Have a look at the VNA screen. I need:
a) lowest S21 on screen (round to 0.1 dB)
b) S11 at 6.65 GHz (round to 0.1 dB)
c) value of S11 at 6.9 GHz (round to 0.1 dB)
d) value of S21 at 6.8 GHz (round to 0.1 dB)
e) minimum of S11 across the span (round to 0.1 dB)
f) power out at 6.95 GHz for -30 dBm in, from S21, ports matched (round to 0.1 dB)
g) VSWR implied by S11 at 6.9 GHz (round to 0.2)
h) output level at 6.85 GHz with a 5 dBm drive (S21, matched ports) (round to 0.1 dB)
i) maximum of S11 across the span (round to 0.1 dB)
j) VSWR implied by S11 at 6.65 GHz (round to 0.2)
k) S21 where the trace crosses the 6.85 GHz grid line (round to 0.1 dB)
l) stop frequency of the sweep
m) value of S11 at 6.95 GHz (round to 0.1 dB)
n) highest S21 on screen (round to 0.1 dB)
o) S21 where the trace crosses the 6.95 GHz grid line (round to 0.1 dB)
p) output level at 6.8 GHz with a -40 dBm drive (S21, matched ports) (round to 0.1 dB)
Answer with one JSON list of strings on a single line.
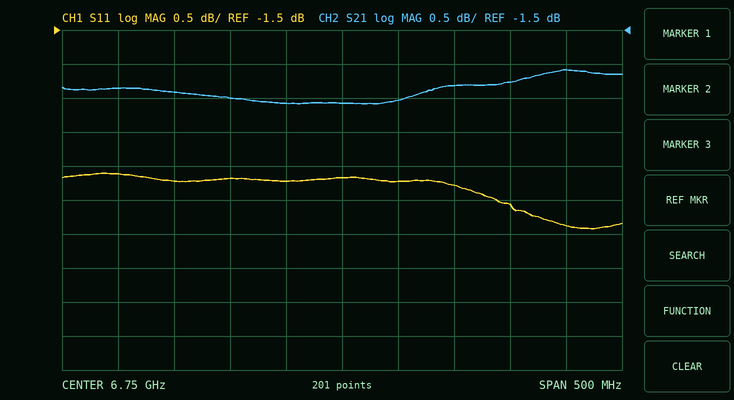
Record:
["-2.6 dB", "-3.7 dB", "-4.1 dB", "-2.5 dB", "-4.4 dB", "-32.1 dBm", "4.4", "2.7 dBm", "-3.6 dB", "4.8", "-2.3 dB", "7 GHz", "-4.4 dB", "-2.1 dB", "-2.1 dB", "-42.5 dBm"]
